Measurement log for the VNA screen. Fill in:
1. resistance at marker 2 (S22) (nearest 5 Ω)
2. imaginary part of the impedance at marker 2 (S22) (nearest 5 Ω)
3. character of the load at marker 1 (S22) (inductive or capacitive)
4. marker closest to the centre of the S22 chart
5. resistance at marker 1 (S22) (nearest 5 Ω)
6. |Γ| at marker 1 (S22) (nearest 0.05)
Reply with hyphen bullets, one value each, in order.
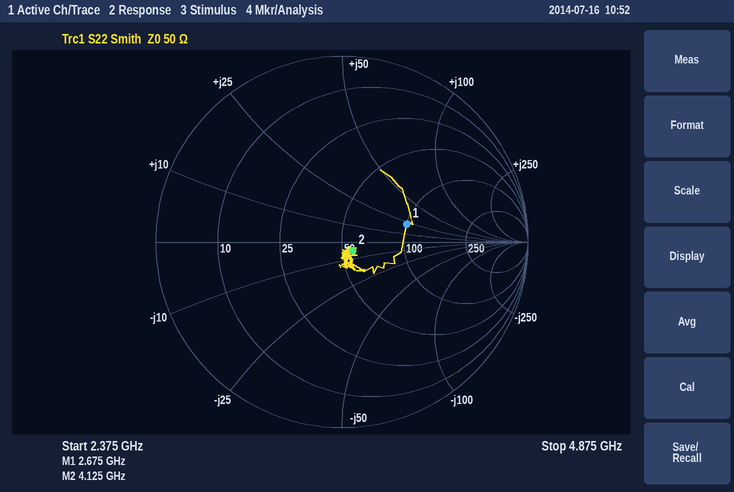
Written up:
- 55 Ω
- -5 Ω
- inductive
- marker 2
- 100 Ω
- 0.35
